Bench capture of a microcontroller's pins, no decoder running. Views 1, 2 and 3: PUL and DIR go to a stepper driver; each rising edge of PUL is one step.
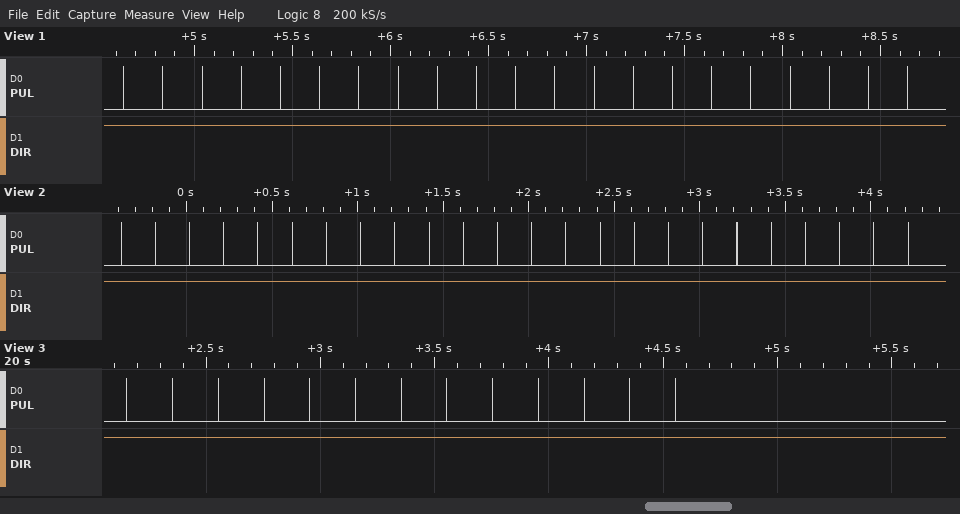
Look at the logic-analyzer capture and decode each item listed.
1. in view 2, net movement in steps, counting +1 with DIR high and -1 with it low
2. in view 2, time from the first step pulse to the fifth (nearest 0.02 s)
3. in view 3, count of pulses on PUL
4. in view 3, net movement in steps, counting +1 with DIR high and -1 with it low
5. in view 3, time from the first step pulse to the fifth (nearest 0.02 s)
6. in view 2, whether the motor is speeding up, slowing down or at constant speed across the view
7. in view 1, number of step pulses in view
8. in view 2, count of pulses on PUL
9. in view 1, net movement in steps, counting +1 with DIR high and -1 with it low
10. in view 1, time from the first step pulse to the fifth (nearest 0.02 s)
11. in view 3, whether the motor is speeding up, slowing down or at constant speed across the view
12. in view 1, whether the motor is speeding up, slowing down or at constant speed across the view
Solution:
+24
0.80 s
13
+13
0.80 s
constant speed
21
24
+21
0.80 s
constant speed
constant speed
